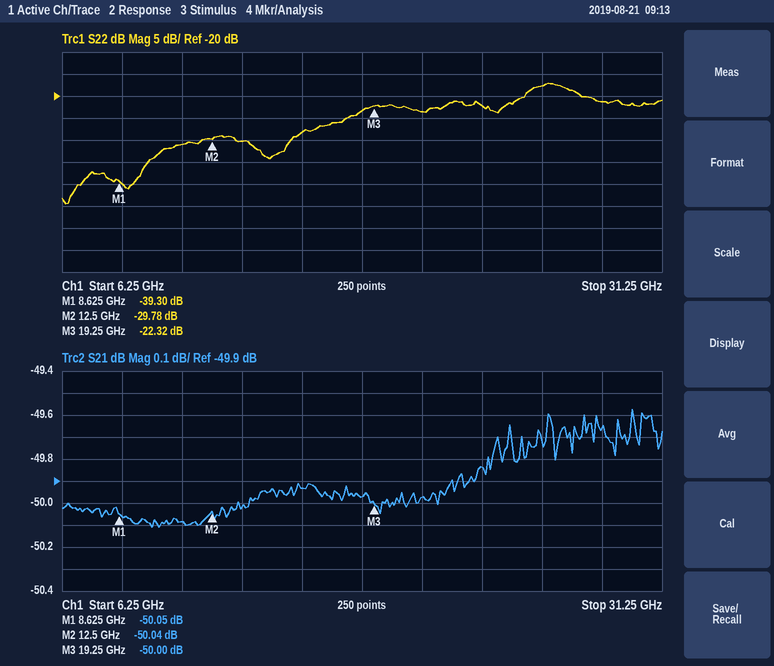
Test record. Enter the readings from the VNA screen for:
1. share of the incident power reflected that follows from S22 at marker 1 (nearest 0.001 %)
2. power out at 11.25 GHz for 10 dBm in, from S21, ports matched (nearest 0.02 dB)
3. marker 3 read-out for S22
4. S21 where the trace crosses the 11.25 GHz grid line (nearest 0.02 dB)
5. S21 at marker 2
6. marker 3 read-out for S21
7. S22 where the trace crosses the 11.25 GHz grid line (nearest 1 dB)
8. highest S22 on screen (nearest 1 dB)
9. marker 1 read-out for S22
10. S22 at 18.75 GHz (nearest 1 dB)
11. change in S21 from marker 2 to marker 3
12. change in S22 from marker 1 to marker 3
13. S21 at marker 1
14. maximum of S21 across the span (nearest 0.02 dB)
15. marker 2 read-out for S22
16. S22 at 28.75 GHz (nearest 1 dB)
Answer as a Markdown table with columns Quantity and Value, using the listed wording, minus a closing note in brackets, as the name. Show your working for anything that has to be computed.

| Quantity | Value |
|---|---|
| share of the incident power reflected that follows from S22 at marker 1 | 10^(-39.3/10) ≈ 0.012 % |
| power out at 11.25 GHz for 10 dBm in, from S21, ports matched | 10 dBm + (-50.08 dB) = -40.08 dBm |
| marker 3 read-out for S22 | -22.32 dB |
| S21 where the trace crosses the 11.25 GHz grid line | -50.08 dB |
| S21 at marker 2 | -50.04 dB |
| marker 3 read-out for S21 | -50.00 dB |
| S22 where the trace crosses the 11.25 GHz grid line | -31 dB |
| highest S22 on screen | -17 dB |
| marker 1 read-out for S22 | -39.30 dB |
| S22 at 18.75 GHz | -23 dB |
| change in S21 from marker 2 to marker 3 | -50 − (-50.04) = 0.04 dB |
| change in S22 from marker 1 to marker 3 | -22.32 − (-39.3) = 16.98 dB |
| S21 at marker 1 | -50.05 dB |
| maximum of S21 across the span | -49.58 dB |
| marker 2 read-out for S22 | -29.78 dB |
| S22 at 28.75 GHz | -21 dB |
